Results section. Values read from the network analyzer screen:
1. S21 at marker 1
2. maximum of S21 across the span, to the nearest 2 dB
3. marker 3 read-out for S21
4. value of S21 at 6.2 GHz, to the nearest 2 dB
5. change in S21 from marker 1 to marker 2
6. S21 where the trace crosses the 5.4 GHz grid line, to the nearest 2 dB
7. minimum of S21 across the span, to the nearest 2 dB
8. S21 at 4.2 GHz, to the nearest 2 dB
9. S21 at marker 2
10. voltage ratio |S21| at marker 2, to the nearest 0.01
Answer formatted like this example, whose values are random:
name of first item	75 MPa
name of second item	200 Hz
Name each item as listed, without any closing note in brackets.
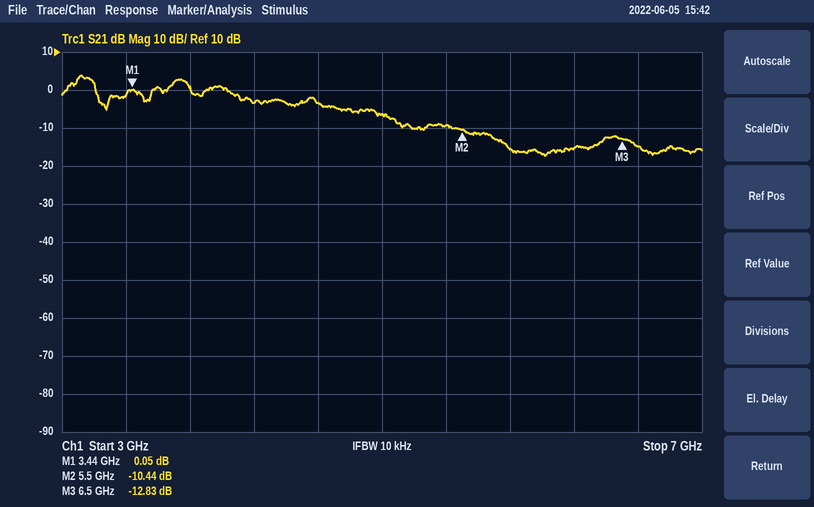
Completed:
S21 at marker 1	0.05 dB
maximum of S21 across the span, to the nearest 2 dB	4 dB
marker 3 read-out for S21	-12.83 dB
value of S21 at 6.2 GHz, to the nearest 2 dB	-16 dB
change in S21 from marker 1 to marker 2	-10.49 dB
S21 where the trace crosses the 5.4 GHz grid line, to the nearest 2 dB	-10 dB
minimum of S21 across the span, to the nearest 2 dB	-18 dB
S21 at 4.2 GHz, to the nearest 2 dB	-4 dB
S21 at marker 2	-10.44 dB
voltage ratio |S21| at marker 2, to the nearest 0.01	0.30
